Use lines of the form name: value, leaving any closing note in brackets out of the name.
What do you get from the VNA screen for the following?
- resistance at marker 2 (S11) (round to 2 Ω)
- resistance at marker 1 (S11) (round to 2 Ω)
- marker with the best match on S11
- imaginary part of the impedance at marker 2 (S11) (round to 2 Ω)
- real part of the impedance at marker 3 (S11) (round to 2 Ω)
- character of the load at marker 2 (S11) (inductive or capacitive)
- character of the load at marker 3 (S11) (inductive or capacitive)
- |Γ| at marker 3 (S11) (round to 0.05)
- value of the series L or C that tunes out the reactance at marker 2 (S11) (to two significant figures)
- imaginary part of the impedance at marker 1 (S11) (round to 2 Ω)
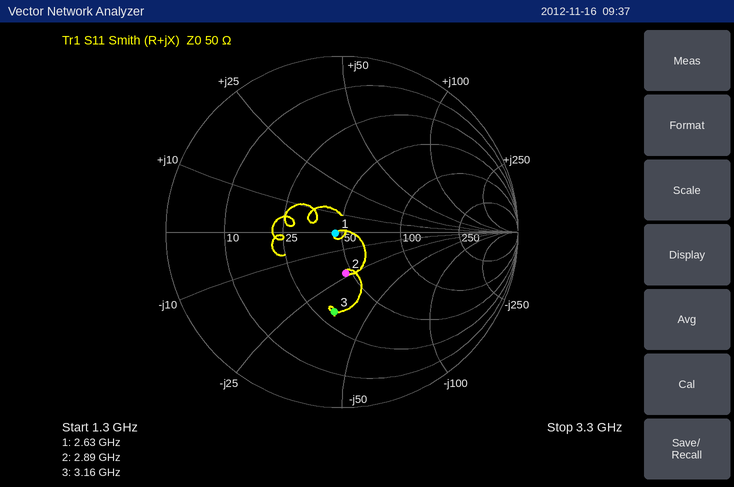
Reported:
resistance at marker 2 (S11): 46 Ω
resistance at marker 1 (S11): 46 Ω
marker with the best match on S11: marker 1
imaginary part of the impedance at marker 2 (S11): -24 Ω
real part of the impedance at marker 3 (S11): 30 Ω
character of the load at marker 2 (S11): capacitive
character of the load at marker 3 (S11): capacitive
|Γ| at marker 3 (S11): 0.45
value of the series L or C that tunes out the reactance at marker 2 (S11): 1.3 nH
imaginary part of the impedance at marker 1 (S11): 0 Ω
